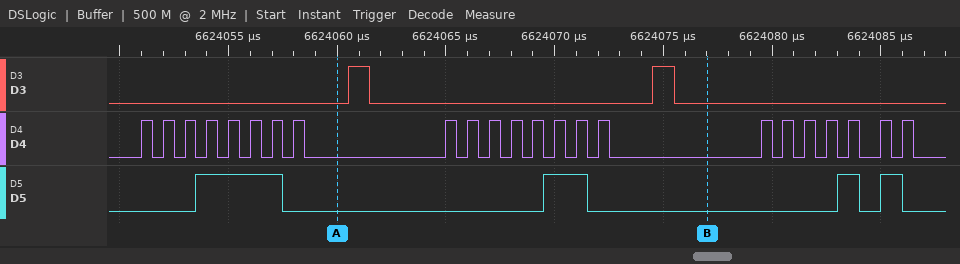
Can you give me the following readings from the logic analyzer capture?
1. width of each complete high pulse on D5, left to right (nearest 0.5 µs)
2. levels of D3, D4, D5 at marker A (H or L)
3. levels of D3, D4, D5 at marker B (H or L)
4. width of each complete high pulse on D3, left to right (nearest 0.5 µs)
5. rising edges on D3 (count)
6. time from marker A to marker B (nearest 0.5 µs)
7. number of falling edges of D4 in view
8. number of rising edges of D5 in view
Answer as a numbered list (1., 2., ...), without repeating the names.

1. 4 µs, 2 µs, 1 µs, 1 µs
2. D3=L, D4=L, D5=L
3. D3=L, D4=L, D5=L
4. 1 µs, 1 µs
5. 2
6. 17 µs
7. 23
8. 4
